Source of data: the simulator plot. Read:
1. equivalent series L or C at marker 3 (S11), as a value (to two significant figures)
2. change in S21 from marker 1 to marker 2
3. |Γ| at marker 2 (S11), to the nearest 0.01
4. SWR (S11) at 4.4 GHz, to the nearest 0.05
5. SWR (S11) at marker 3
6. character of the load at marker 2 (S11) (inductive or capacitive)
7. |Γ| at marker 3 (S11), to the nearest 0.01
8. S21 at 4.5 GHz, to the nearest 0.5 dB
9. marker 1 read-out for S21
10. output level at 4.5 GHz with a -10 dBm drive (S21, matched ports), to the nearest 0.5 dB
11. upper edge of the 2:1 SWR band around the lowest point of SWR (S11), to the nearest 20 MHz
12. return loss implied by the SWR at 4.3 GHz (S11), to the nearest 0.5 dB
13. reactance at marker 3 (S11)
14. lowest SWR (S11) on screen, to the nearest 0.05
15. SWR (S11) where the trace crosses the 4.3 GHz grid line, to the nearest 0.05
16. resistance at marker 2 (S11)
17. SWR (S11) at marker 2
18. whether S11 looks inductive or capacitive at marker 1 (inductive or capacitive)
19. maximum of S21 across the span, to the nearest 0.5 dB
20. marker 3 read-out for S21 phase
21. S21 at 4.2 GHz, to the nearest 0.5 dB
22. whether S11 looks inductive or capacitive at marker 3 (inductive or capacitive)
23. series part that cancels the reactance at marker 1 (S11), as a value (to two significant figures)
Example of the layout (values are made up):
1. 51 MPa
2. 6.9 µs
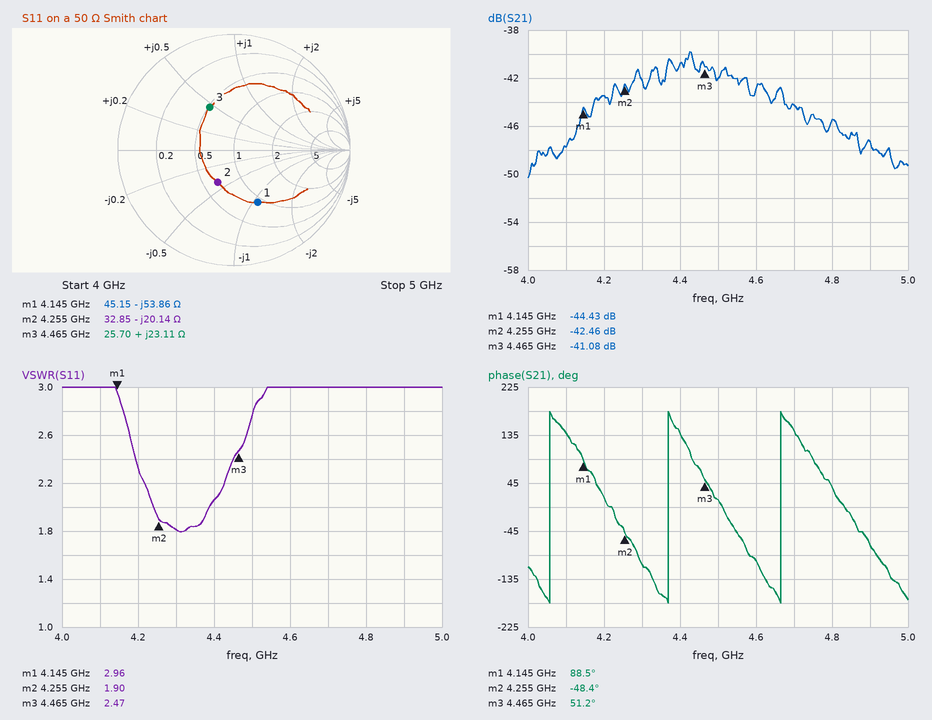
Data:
1. 820 pH
2. 1.97 dB
3. 0.31
4. 2.05
5. 2.47
6. capacitive
7. 0.42
8. -42.0 dB
9. -44.43 dB
10. -52.0 dBm
11. 4.38 GHz
12. 11.0 dB
13. +23.11 Ω
14. 1.80
15. 1.80
16. 32.85 Ω
17. 1.90
18. capacitive
19. -40.0 dB
20. 51.2°
21. -43.5 dB
22. inductive
23. 2.1 nH
